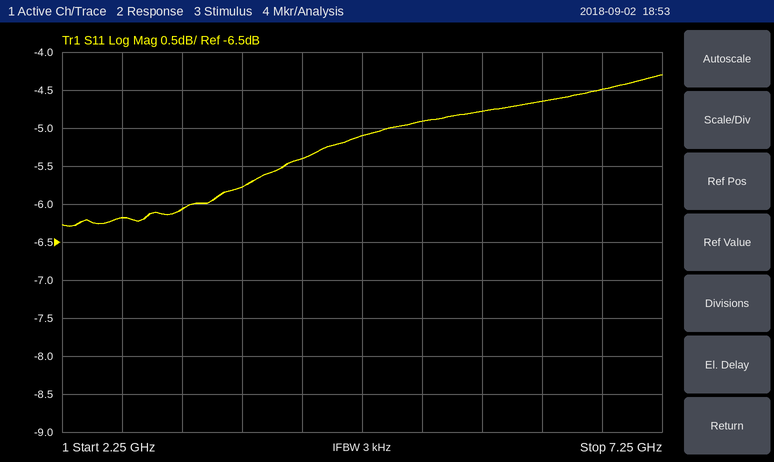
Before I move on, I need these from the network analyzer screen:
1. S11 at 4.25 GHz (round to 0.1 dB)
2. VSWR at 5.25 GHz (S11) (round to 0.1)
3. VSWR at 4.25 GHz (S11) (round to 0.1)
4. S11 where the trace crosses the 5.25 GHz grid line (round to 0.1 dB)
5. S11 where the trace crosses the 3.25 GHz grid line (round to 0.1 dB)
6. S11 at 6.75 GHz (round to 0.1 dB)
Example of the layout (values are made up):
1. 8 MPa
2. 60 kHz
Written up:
1. -5.4 dB
2. 3.6
3. 3.3
4. -4.9 dB
5. -6.1 dB
6. -4.5 dB
